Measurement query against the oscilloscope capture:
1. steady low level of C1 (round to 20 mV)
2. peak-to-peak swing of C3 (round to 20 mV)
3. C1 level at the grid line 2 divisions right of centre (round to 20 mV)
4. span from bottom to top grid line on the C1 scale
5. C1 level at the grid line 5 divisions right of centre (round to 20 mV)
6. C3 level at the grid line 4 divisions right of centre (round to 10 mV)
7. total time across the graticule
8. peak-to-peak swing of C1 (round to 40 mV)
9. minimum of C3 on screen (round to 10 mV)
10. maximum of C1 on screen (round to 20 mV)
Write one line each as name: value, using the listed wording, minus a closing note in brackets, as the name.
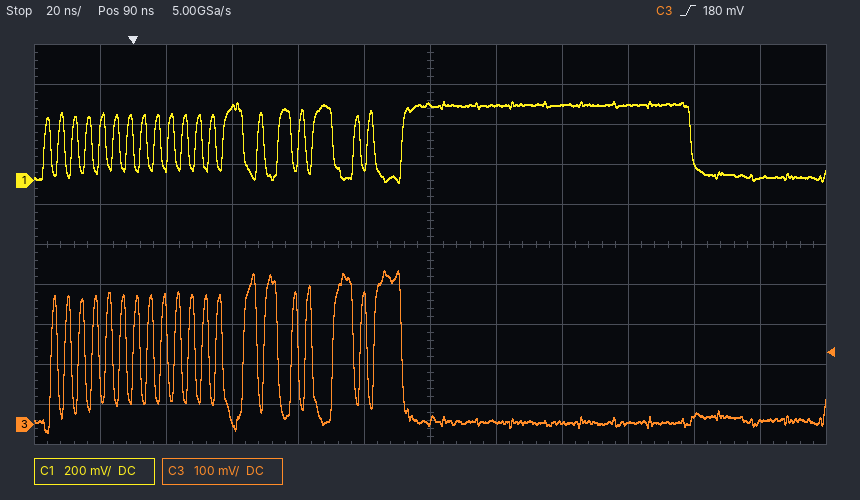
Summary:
steady low level of C1: 20 mV
peak-to-peak swing of C3: 400 mV
C1 level at the grid line 2 divisions right of centre: 380 mV
span from bottom to top grid line on the C1 scale: 2 V
C1 level at the grid line 5 divisions right of centre: 20 mV
C3 level at the grid line 4 divisions right of centre: 20 mV
total time across the graticule: 240 ns
peak-to-peak swing of C1: 400 mV
minimum of C3 on screen: -20 mV
maximum of C1 on screen: 400 mV
